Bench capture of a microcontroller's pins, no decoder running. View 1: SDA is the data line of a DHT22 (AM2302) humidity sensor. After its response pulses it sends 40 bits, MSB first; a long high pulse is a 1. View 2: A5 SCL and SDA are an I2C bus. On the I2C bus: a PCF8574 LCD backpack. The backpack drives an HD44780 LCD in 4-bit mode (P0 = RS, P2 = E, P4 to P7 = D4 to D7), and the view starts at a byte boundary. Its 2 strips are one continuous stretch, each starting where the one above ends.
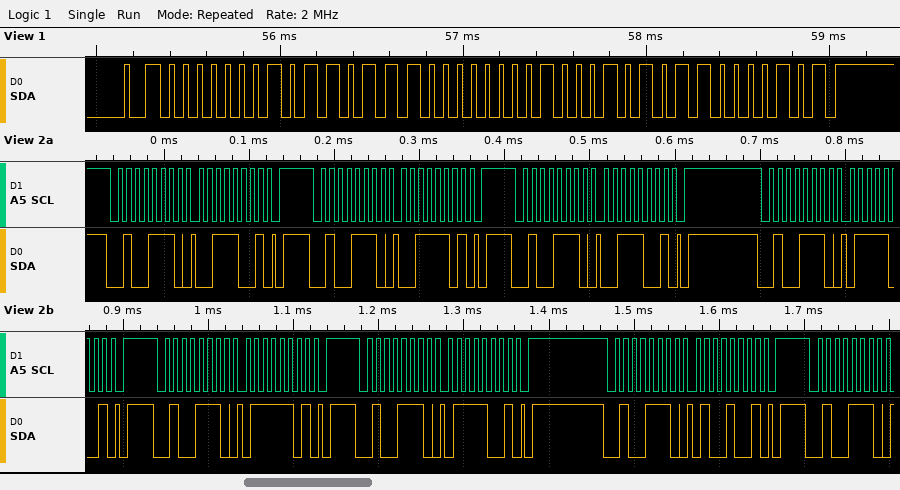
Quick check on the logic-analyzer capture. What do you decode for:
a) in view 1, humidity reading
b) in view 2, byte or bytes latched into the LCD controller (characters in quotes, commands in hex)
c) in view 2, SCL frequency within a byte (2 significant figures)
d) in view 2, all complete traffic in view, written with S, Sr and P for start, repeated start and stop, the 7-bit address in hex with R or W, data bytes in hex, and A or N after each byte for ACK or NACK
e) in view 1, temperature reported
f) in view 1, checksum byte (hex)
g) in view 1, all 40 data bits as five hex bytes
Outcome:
36.6 %
'7'
100 kHz
S 27W A 39 A P S 27W A 3D A P S 27W A 39 A P S 27W A 79 A P S 27W A 7D A P S 27W A 79 A P S 27W A 49 A P S 27W A
27.7 °C
0x85
01 6E 01 15 85
